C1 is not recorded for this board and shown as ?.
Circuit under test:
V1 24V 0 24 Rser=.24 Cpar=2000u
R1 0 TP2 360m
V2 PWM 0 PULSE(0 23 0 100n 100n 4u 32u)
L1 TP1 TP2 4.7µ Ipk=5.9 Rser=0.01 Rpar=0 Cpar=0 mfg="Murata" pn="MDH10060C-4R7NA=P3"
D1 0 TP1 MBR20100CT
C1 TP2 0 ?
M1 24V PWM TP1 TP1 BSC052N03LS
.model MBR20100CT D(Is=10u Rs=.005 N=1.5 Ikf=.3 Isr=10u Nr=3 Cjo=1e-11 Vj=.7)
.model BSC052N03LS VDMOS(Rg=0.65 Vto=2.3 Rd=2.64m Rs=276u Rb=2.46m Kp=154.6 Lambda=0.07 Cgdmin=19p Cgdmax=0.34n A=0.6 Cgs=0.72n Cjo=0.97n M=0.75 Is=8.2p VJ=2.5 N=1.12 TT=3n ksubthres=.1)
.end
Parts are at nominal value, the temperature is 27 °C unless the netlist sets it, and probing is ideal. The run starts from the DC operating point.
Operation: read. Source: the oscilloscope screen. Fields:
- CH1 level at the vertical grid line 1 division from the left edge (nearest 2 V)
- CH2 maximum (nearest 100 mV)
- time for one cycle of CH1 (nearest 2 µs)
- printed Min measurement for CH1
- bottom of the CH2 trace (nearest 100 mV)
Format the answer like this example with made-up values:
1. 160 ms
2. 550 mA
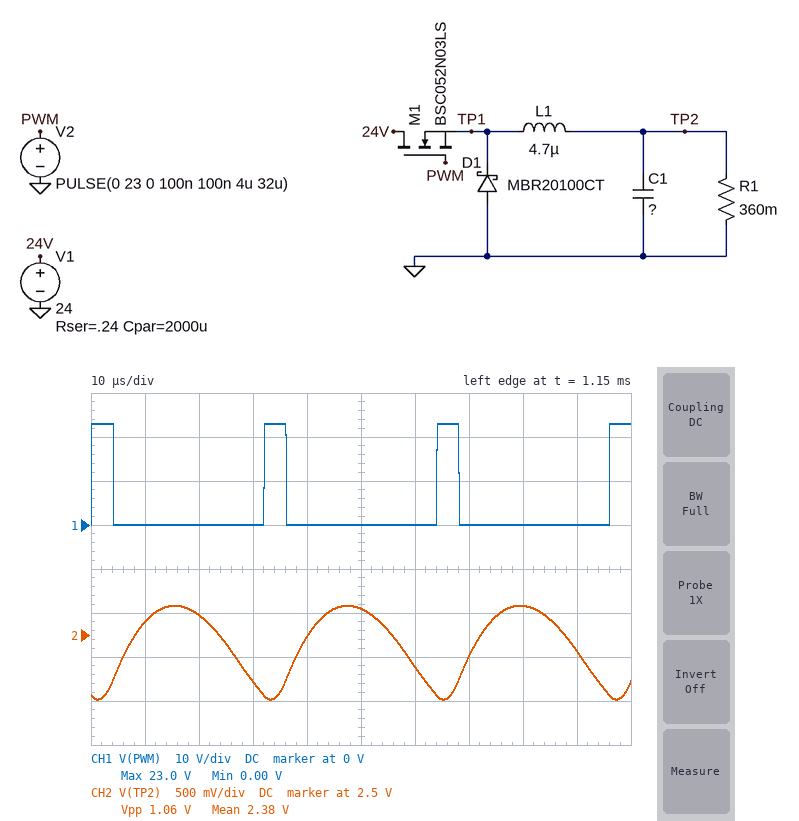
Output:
1. 0 V
2. 2.8 V
3. 32 µs
4. 0.00 V
5. 1.8 V
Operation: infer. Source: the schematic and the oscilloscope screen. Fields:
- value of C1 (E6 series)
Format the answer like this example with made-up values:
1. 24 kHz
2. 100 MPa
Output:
1. 68 µF
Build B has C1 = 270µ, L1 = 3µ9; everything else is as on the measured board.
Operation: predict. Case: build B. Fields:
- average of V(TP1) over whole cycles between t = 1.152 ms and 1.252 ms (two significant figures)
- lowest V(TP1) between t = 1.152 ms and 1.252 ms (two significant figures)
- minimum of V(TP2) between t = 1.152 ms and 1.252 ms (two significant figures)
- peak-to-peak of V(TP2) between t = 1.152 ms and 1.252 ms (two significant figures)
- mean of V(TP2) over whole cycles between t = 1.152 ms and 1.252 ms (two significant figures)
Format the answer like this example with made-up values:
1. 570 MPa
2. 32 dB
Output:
1. 2.7 V
2. -820 mV
3. 2.4 V
4. 320 mV
5. 2.6 V
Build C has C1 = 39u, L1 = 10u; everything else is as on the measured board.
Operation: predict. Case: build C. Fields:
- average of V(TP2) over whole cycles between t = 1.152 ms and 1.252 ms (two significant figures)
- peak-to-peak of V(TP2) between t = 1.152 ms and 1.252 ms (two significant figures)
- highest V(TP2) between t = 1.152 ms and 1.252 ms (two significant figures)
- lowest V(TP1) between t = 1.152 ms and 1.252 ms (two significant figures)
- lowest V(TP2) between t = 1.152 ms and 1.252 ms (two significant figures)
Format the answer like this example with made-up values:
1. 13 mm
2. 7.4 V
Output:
1. 2.0 V
2. 770 mV
3. 2.3 V
4. -720 mV
5. 1.5 V
